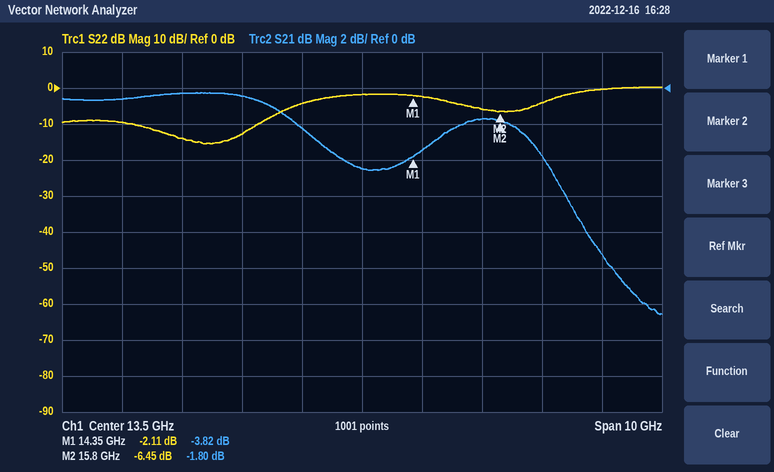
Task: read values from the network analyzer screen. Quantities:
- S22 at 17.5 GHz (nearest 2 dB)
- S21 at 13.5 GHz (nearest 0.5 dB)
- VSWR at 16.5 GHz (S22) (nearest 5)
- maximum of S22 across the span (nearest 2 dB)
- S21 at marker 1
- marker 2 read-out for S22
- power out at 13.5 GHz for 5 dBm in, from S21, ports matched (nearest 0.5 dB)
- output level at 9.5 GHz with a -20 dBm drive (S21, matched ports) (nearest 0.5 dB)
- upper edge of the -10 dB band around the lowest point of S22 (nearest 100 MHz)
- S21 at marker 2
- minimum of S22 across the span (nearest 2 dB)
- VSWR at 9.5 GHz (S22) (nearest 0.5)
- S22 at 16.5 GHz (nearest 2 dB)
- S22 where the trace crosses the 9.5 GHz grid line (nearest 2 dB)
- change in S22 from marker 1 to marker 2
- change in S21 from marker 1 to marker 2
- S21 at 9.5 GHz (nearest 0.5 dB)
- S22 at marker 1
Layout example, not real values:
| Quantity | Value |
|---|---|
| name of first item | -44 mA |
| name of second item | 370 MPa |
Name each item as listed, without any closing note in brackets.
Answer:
| Quantity | Value |
|---|---|
| S22 at 17.5 GHz | 0 dB |
| S21 at 13.5 GHz | -4.5 dB |
| VSWR at 16.5 GHz (S22) | 5 |
| maximum of S22 across the span | 0 dB |
| S21 at marker 1 | -3.82 dB |
| marker 2 read-out for S22 | -6.45 dB |
| power out at 13.5 GHz for 5 dBm in, from S21, ports matched | 0.5 dBm |
| output level at 9.5 GHz with a -20 dBm drive (S21, matched ports) | -20.5 dBm |
| upper edge of the -10 dB band around the lowest point of S22 | 11.8 GHz |
| S21 at marker 2 | -1.80 dB |
| minimum of S22 across the span | -16 dB |
| VSWR at 9.5 GHz (S22) | 2.0 |
| S22 at 16.5 GHz | -4 dB |
| S22 where the trace crosses the 9.5 GHz grid line | -10 dB |
| change in S22 from marker 1 to marker 2 | -4.34 dB |
| change in S21 from marker 1 to marker 2 | 2.02 dB |
| S21 at 9.5 GHz | -0.5 dB |
| S22 at marker 1 | -2.11 dB |
